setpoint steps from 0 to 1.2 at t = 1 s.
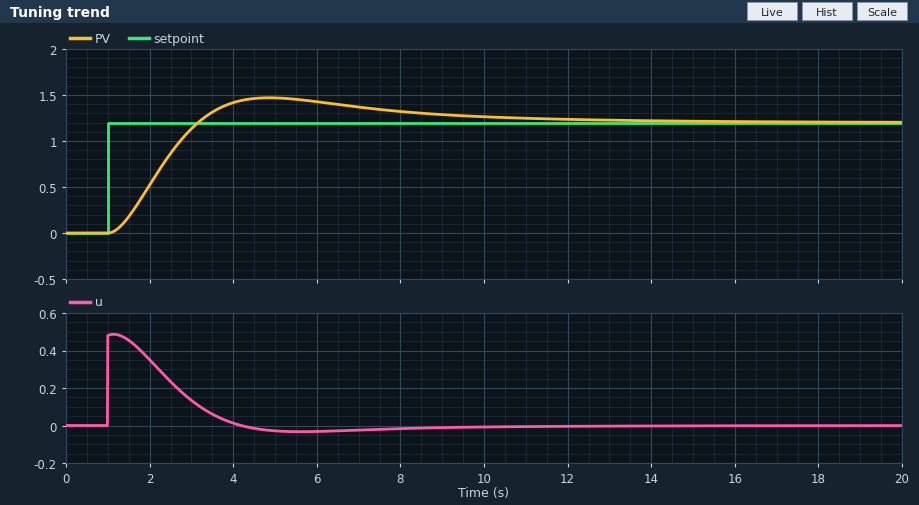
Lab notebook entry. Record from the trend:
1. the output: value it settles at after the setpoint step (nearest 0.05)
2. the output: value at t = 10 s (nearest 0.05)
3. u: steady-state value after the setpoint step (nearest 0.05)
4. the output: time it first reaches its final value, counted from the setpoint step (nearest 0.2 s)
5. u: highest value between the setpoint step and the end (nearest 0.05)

1.20
1.25
0.00
2.2 s
0.50
